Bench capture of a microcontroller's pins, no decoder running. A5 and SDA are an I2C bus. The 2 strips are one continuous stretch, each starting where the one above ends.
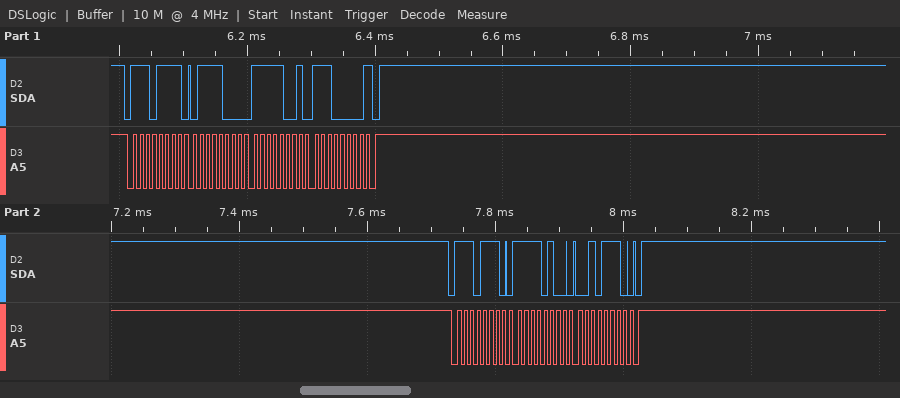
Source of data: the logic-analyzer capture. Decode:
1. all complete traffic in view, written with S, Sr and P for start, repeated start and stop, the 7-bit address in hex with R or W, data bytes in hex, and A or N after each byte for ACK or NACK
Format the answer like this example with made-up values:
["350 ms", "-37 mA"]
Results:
["S 77R A 78 A F9 A E0 N P S 77W A F4 A 2E A P"]
